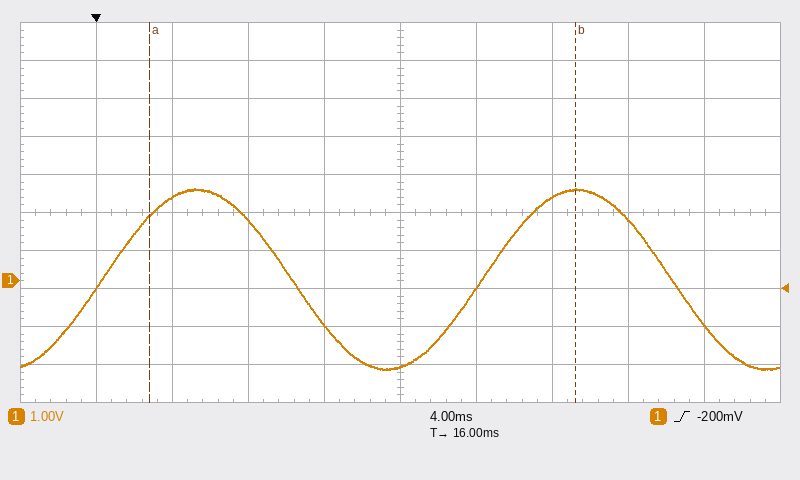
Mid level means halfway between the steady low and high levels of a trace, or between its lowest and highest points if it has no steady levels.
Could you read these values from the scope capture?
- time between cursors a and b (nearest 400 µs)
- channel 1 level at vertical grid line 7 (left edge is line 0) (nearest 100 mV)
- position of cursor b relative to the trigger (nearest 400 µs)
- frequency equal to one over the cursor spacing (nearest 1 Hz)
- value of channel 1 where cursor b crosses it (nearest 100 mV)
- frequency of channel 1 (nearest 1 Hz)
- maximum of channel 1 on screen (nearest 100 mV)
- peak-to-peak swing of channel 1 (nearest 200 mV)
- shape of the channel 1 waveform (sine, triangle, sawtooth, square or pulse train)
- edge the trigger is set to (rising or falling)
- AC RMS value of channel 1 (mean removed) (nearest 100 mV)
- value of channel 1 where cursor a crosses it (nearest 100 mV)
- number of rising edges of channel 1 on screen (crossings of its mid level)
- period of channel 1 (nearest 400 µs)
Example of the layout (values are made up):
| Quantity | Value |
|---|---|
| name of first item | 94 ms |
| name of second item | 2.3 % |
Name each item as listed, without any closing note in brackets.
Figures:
| Quantity | Value |
|---|---|
| time between cursors a and b | 22.4 ms |
| channel 1 level at vertical grid line 7 (left edge is line 0) | 2.2 V |
| position of cursor b relative to the trigger | +25.2 ms |
| frequency equal to one over the cursor spacing | 45 Hz |
| value of channel 1 where cursor b crosses it | 2.4 V |
| frequency of channel 1 | 50 Hz |
| maximum of channel 1 on screen | 2.4 V |
| peak-to-peak swing of channel 1 | 4.8 V |
| shape of the channel 1 waveform | sine |
| edge the trigger is set to | rising |
| AC RMS value of channel 1 (mean removed) | 1.7 V |
| value of channel 1 where cursor a crosses it | 1.7 V |
| number of rising edges of channel 1 on screen | 2 |
| period of channel 1 | 20.0 ms |
